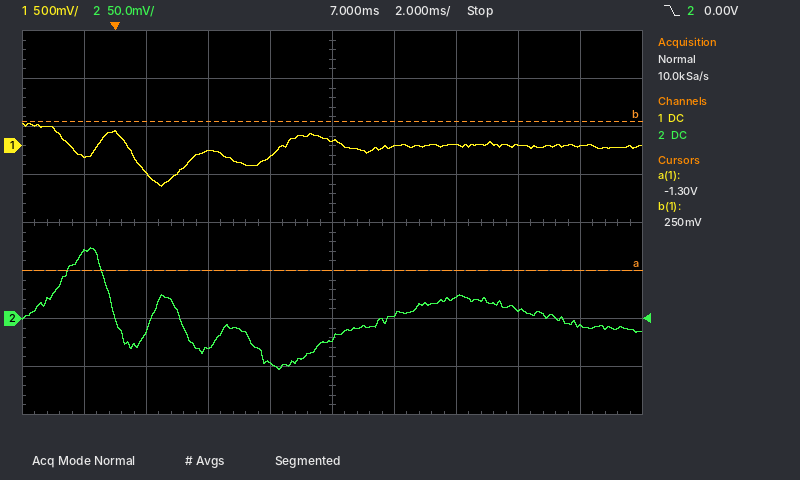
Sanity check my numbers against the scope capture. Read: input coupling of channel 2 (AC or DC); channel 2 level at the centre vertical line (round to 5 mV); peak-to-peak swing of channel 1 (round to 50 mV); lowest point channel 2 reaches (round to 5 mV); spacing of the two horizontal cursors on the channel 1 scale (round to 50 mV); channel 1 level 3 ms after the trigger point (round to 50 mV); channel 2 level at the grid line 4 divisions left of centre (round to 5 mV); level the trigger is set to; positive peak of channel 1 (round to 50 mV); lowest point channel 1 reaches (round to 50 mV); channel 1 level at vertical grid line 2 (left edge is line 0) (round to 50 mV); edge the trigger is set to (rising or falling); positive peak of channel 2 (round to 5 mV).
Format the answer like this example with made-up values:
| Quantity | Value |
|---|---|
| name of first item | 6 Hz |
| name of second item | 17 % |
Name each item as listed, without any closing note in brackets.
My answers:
| Quantity | Value |
|---|---|
| input coupling of channel 2 | DC |
| channel 2 level at the centre vertical line | -20 mV |
| peak-to-peak swing of channel 1 | 650 mV |
| lowest point channel 2 reaches | -55 mV |
| spacing of the two horizontal cursors on the channel 1 scale | 1.55 V |
| channel 1 level 3 ms after the trigger point | -50 mV |
| channel 2 level at the grid line 4 divisions left of centre | 70 mV |
| level the trigger is set to | 0.00 V |
| positive peak of channel 1 | 250 mV |
| lowest point channel 1 reaches | -400 mV |
| channel 1 level at vertical grid line 2 (left edge is line 0) | -300 mV |
| edge the trigger is set to | falling |
| positive peak of channel 2 | 75 mV |
